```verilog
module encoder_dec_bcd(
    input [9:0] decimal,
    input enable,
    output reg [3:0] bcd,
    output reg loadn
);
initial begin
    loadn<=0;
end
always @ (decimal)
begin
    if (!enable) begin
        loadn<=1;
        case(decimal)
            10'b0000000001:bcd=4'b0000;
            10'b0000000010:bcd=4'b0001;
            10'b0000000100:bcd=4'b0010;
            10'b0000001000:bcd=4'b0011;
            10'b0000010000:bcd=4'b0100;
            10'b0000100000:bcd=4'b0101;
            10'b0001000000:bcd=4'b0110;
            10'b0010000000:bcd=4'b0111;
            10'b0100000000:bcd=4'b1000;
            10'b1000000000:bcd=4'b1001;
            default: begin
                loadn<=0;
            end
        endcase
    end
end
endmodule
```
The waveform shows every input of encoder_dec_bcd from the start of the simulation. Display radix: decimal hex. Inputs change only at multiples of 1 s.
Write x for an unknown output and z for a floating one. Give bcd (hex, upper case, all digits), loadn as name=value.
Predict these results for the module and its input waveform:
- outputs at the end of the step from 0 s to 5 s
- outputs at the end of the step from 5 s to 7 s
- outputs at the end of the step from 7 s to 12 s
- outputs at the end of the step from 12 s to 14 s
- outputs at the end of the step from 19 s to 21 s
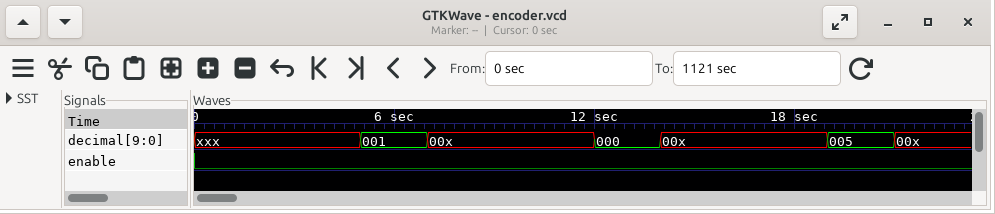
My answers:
bcd=x, loadn=0
bcd=0, loadn=1
bcd=0, loadn=0
bcd=0, loadn=0
bcd=0, loadn=0
